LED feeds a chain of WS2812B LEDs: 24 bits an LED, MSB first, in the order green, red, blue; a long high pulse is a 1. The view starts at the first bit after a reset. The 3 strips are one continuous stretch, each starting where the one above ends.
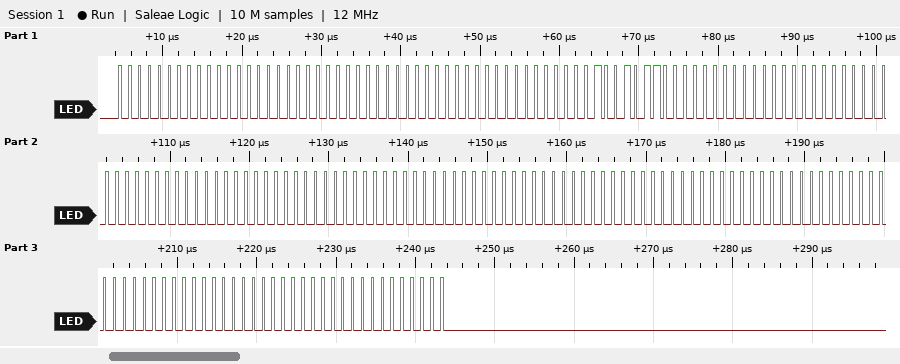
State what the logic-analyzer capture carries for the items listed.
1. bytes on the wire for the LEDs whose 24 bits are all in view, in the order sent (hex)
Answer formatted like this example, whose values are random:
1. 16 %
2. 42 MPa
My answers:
1. 00 00 00 00 00 00 96 00 00 00 00 00 00 00 00 00 00 00 00 00 00 00 00 00
